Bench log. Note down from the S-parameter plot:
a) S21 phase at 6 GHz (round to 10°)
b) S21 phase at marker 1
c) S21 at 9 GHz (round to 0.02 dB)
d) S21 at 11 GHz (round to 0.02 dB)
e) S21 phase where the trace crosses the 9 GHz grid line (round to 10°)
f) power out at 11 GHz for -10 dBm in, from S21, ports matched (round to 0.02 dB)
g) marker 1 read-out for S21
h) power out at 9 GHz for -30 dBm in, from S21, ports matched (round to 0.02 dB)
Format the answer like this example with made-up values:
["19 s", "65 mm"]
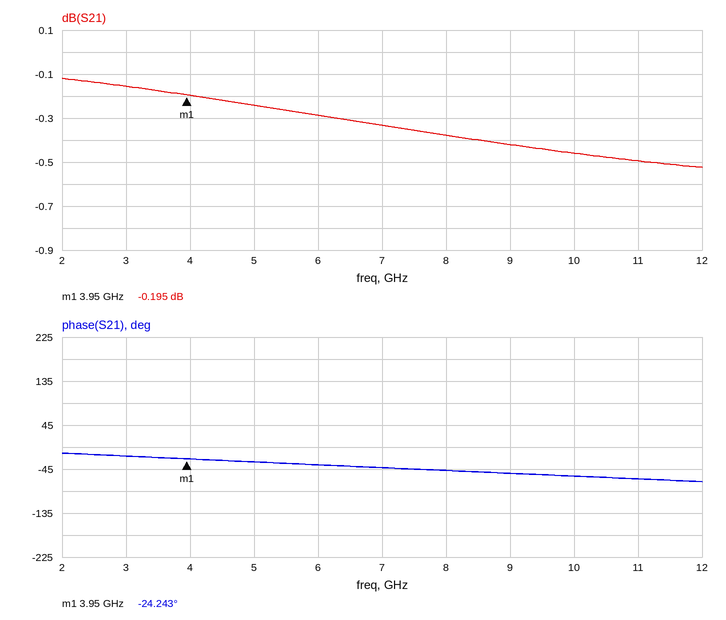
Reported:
["-40°", "-24.243°", "-0.42 dB", "-0.50 dB", "-50°", "-10.50 dBm", "-0.195 dB", "-30.42 dBm"]
